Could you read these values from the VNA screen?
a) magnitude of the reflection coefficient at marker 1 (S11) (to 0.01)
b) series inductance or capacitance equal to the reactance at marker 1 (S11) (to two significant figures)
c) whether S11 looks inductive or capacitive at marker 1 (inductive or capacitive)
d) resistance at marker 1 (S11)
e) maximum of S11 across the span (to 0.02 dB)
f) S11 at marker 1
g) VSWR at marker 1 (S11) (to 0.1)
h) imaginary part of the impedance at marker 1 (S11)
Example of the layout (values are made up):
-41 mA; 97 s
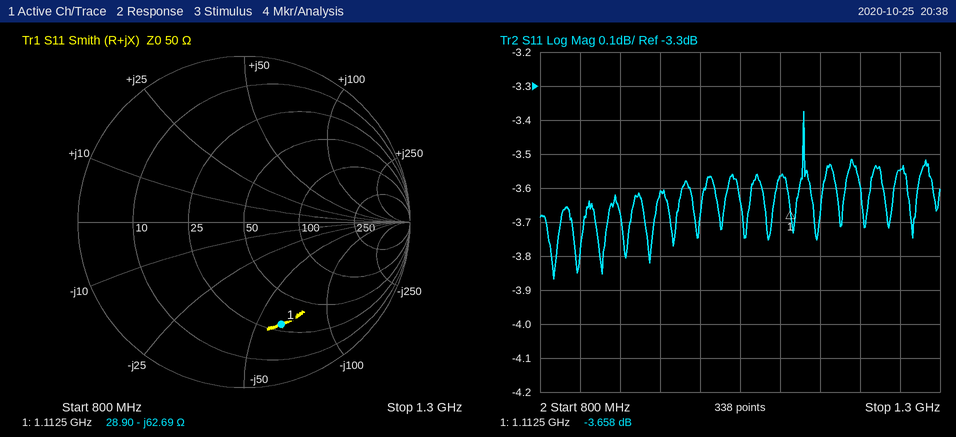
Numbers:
0.66; 2.3 pF; capacitive; 28.90 Ω; -3.38 dB; -3.658 dB; 4.8; -62.69 Ω
